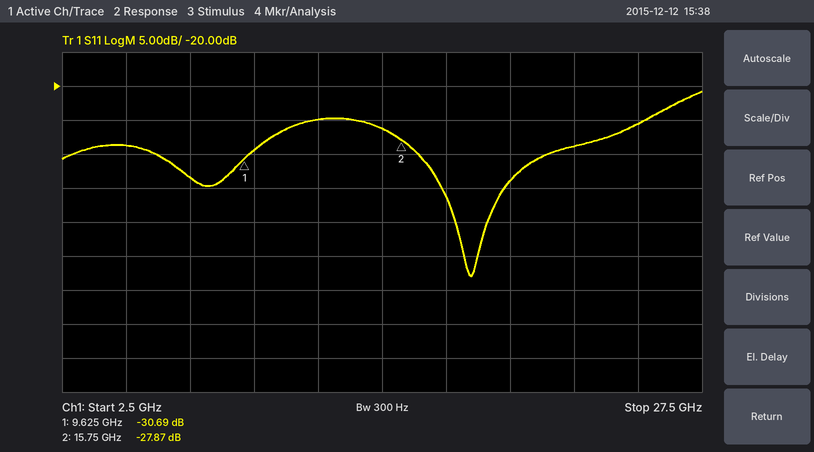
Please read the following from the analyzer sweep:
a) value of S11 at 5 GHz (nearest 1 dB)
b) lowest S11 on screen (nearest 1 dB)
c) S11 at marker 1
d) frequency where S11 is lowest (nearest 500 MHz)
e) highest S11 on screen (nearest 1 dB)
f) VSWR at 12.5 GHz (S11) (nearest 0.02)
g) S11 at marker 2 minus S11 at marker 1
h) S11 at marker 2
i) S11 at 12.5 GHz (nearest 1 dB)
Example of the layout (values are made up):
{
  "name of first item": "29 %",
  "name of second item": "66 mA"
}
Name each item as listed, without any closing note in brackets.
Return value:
{
  "value of S11 at 5 GHz": "-29 dB",
  "lowest S11 on screen": "-48 dB",
  "S11 at marker 1": "-30.69 dB",
  "frequency where S11 is lowest": "18.5 GHz",
  "highest S11 on screen": "-21 dB",
  "VSWR at 12.5 GHz (S11)": "1.12",
  "S11 at marker 2 minus S11 at marker 1": "2.82 dB",
  "S11 at marker 2": "-27.87 dB",
  "S11 at 12.5 GHz": "-25 dB"
}
